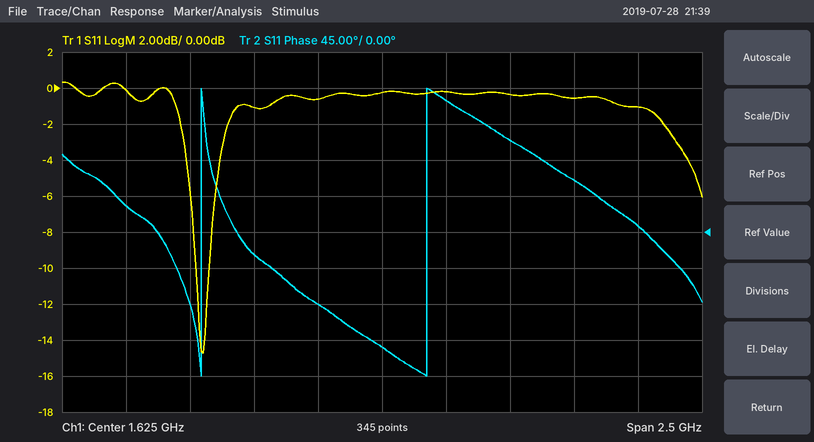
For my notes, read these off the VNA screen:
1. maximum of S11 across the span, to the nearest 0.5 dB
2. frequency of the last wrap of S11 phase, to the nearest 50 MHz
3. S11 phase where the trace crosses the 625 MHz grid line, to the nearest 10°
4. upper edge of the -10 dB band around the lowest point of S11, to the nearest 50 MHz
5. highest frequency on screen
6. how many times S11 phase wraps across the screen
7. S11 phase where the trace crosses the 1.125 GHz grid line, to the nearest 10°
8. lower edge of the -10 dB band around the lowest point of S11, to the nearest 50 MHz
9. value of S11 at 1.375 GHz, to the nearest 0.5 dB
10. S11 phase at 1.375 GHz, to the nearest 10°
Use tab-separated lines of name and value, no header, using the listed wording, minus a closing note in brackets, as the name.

maximum of S11 across the span, to the nearest 0.5 dB	0.5 dB
frequency of the last wrap of S11 phase, to the nearest 50 MHz	1.80 GHz
S11 phase where the trace crosses the 625 MHz grid line, to the nearest 10°	30°
upper edge of the -10 dB band around the lowest point of S11, to the nearest 50 MHz	950 MHz
highest frequency on screen	2.875 GHz
how many times S11 phase wraps across the screen	2
S11 phase where the trace crosses the 1.125 GHz grid line, to the nearest 10°	-30°
lower edge of the -10 dB band around the lowest point of S11, to the nearest 50 MHz	900 MHz
value of S11 at 1.375 GHz, to the nearest 0.5 dB	-0.5 dB
S11 phase at 1.375 GHz, to the nearest 10°	-90°
